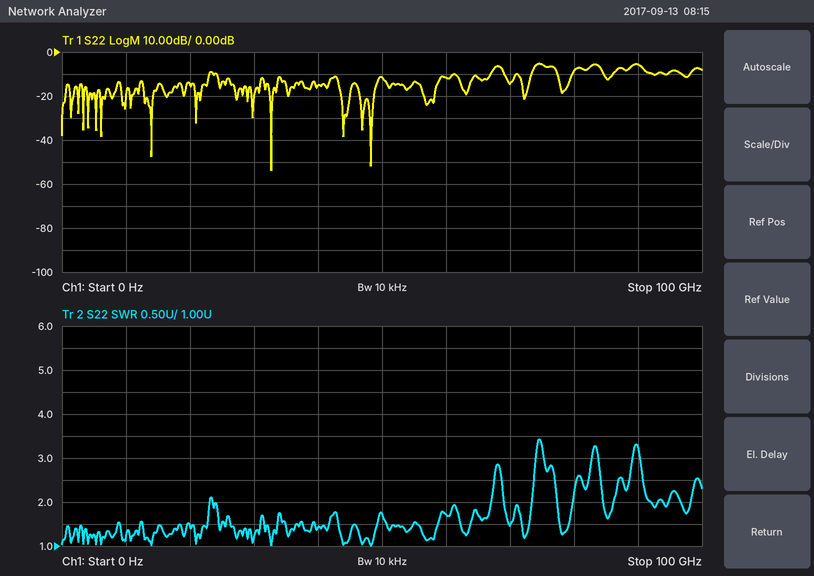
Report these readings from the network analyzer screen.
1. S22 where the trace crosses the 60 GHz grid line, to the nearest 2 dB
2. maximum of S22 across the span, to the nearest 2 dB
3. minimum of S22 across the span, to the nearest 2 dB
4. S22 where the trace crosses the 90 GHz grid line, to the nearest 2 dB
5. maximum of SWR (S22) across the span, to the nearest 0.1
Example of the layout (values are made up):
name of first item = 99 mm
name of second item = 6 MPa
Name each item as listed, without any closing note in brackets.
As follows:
S22 where the trace crosses the 60 GHz grid line, to the nearest 2 dB = -12 dB
maximum of S22 across the span, to the nearest 2 dB = -6 dB
minimum of S22 across the span, to the nearest 2 dB = -54 dB
S22 where the trace crosses the 90 GHz grid line, to the nearest 2 dB = -6 dB
maximum of SWR (S22) across the span, to the nearest 0.1 = 3.4
